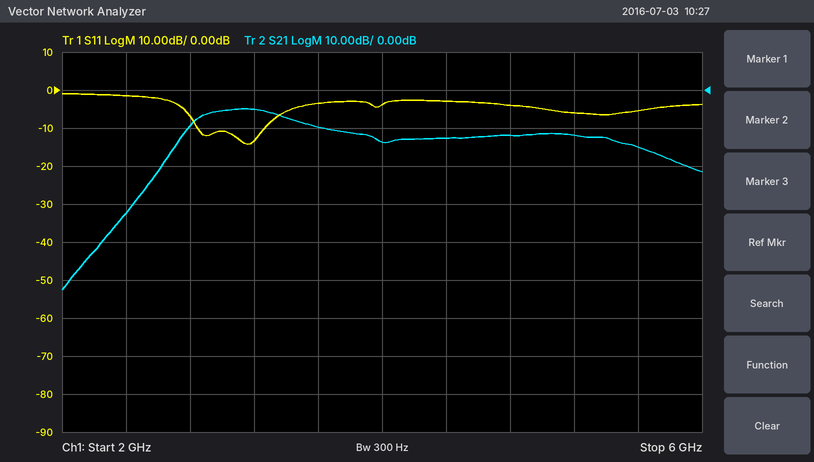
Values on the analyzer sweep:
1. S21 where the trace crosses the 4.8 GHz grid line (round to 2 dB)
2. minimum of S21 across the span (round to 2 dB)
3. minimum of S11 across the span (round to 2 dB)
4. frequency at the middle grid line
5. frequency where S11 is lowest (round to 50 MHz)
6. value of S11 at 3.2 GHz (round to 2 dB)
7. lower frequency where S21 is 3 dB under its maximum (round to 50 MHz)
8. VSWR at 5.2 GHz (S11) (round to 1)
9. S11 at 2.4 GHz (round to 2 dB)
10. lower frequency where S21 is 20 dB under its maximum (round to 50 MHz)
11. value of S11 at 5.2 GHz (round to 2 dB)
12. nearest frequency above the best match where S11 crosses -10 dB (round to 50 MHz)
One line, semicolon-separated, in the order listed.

-12 dB; -52 dB; -14 dB; 4 GHz; 3.15 GHz; -14 dB; 2.85 GHz; 3; -2 dB; 2.55 GHz; -6 dB; 3.25 GHz
